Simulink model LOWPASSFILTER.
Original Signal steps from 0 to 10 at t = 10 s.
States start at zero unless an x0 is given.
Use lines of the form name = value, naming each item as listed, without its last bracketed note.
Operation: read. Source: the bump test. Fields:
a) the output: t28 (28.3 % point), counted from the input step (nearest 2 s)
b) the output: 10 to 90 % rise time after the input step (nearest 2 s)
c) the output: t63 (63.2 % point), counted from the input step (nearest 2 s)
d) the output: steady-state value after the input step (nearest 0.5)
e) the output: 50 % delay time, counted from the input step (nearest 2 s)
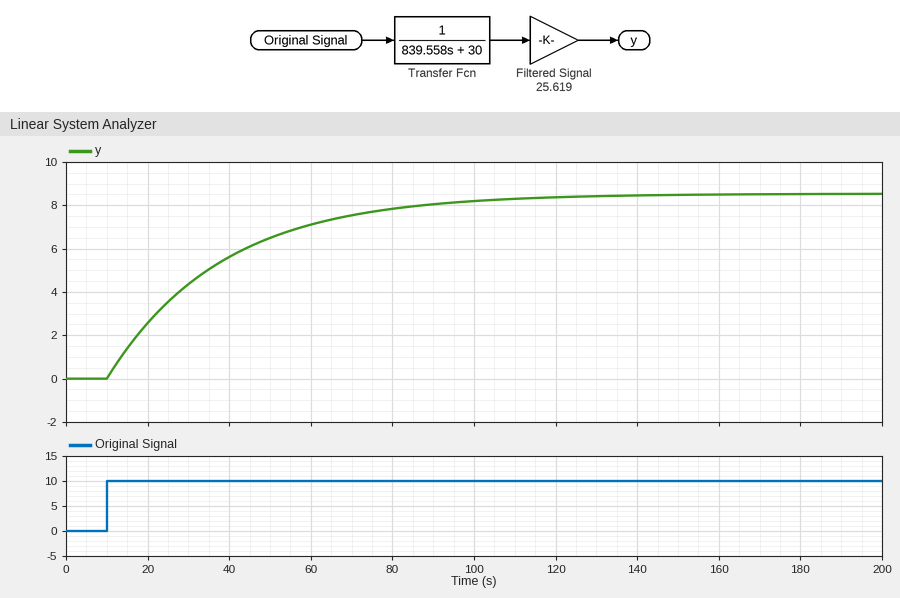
the output: t28 (28.3 % point), counted from the input step = 10 s
the output: 10 to 90 % rise time after the input step = 62 s
the output: t63 (63.2 % point), counted from the input step = 28 s
the output: steady-state value after the input step = 8.5
the output: 50 % delay time, counted from the input step = 20 s
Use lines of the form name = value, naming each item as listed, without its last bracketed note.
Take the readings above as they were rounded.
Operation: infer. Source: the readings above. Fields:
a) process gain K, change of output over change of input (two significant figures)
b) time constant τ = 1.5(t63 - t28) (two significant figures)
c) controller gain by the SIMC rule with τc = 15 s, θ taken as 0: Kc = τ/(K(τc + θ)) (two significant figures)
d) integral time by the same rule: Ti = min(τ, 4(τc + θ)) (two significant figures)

process gain K, change of output over change of input = 0.85
time constant τ = 1.5(t63 - t28) = 27 s
controller gain by the SIMC rule with τc = 15 s, θ taken as 0: Kc = τ/(K(τc + θ)) = 2.1
integral time by the same rule: Ti = min(τ, 4(τc + θ)) = 27 s
